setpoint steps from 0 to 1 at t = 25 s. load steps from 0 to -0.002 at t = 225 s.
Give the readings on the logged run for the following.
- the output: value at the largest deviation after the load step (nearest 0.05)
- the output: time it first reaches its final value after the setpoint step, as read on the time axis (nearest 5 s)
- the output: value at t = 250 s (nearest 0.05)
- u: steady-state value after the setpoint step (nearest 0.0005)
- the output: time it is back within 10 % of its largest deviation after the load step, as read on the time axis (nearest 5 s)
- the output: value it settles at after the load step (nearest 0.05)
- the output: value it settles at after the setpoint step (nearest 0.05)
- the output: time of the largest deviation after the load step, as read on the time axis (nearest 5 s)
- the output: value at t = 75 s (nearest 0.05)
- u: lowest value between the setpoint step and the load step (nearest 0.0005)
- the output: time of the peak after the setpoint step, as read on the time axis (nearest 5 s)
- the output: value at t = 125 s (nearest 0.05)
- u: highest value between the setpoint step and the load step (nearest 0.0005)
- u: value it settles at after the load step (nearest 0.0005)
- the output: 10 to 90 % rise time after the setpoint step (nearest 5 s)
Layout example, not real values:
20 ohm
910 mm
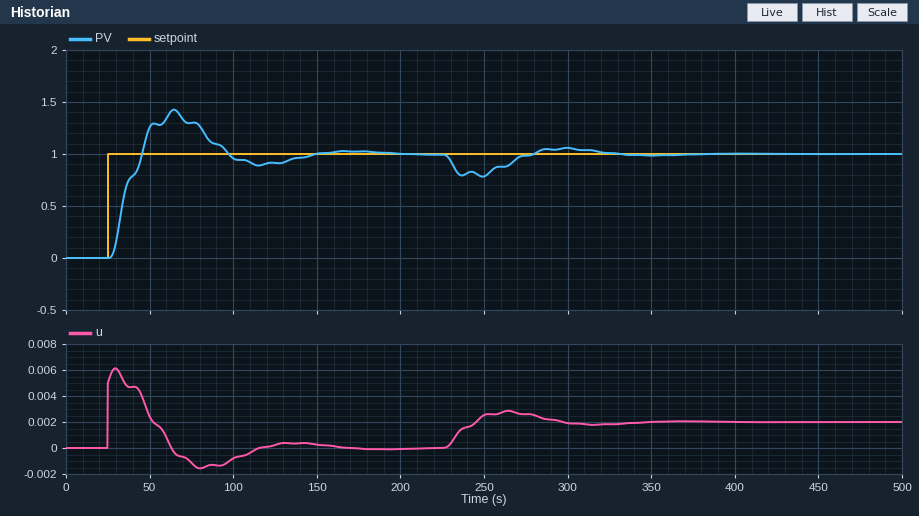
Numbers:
0.80
45 s
0.80
0.0000
320 s
1.00
1.00
250 s
1.30
-0.0015
65 s
0.90
0.0060
0.0020
15 s
